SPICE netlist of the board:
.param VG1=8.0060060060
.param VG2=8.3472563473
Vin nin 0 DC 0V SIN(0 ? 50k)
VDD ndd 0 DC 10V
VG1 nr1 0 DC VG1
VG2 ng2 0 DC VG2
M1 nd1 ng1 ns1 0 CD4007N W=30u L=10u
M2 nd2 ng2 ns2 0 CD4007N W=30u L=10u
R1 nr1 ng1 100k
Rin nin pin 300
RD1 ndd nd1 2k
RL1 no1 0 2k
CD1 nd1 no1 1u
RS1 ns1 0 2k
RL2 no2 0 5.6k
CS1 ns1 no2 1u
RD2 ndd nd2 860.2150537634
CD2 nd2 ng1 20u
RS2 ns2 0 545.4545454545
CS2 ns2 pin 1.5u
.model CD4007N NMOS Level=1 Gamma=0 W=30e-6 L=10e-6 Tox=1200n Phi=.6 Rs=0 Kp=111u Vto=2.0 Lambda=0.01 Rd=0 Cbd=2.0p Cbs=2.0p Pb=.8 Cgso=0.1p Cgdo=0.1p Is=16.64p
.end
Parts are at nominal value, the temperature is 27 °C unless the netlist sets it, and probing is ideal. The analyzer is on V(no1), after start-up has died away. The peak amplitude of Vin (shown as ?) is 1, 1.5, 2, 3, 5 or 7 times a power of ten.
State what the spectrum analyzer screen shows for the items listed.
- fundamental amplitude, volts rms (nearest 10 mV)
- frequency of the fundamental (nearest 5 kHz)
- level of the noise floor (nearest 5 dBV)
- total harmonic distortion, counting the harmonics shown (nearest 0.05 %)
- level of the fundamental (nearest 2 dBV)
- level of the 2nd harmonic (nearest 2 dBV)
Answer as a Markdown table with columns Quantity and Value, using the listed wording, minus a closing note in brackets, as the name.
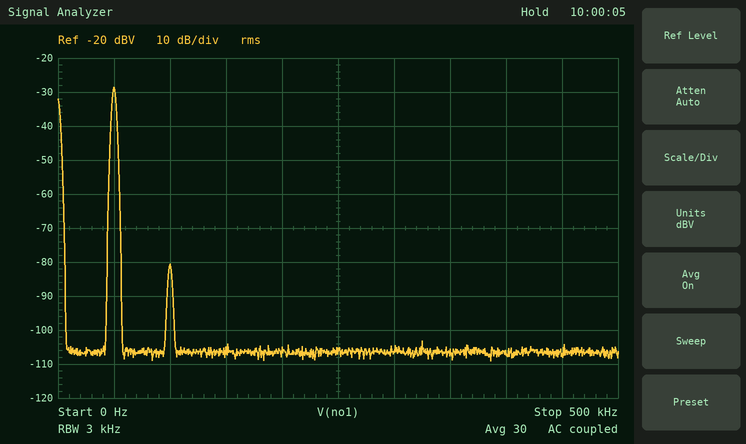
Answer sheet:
| Quantity | Value |
|---|---|
| fundamental amplitude, volts rms | 40 mV |
| frequency of the fundamental | 50 kHz |
| level of the noise floor | -105 dBV |
| total harmonic distortion, counting the harmonics shown | 0.25 % |
| level of the fundamental | -28 dBV |
| level of the 2nd harmonic | -80 dBV |
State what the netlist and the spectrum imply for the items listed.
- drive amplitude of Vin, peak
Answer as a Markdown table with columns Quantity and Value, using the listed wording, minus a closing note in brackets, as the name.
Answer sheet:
| Quantity | Value |
|---|---|
| drive amplitude of Vin, peak | 200 mV |
